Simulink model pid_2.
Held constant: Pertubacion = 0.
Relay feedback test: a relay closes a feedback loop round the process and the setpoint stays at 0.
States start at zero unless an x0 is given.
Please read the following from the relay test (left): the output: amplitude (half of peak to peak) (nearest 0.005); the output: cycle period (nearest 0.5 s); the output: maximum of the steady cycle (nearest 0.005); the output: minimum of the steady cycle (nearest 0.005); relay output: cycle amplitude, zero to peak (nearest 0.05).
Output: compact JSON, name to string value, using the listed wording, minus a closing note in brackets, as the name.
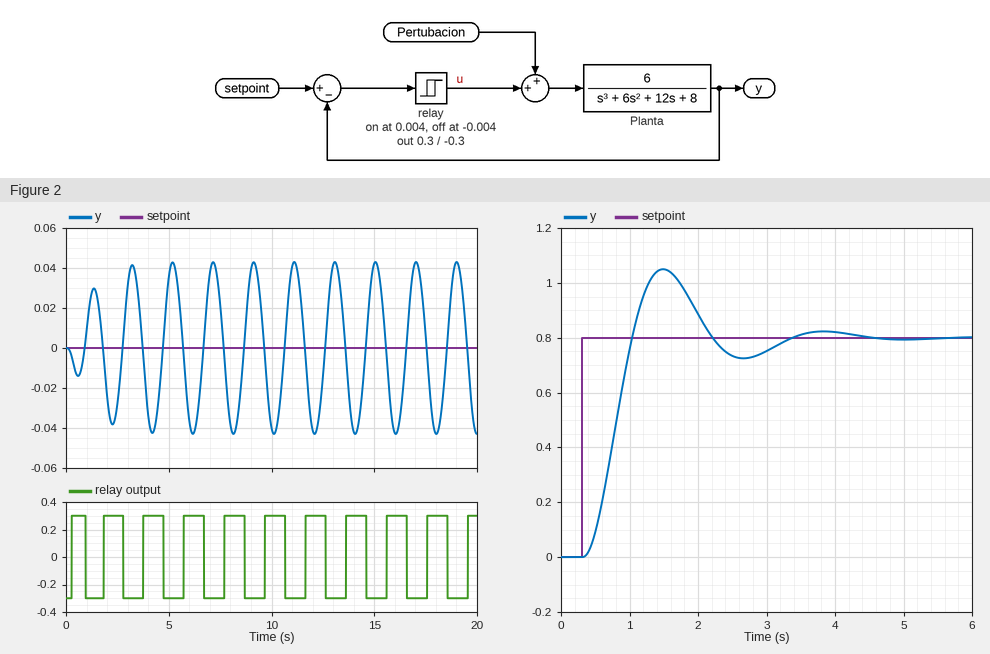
{"the output: amplitude (half of peak to peak)": "0.045", "the output: cycle period": "2.0 s", "the output: maximum of the steady cycle": "0.045", "the output: minimum of the steady cycle": "-0.045", "relay output: cycle amplitude, zero to peak": "0.30"}
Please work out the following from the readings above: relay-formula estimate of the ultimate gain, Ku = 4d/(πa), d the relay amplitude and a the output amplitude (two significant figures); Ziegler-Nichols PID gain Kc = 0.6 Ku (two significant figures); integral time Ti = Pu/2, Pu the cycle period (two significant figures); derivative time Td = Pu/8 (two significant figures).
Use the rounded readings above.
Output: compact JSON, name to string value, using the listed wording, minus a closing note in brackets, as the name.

{"relay-formula estimate of the ultimate gain, Ku = 4d/(πa), d the relay amplitude and a the output amplitude": "8.5", "Ziegler-Nichols PID gain Kc = 0.6 Ku": "5.1", "integral time Ti = Pu/2, Pu the cycle period": "1.0 s", "derivative time Td = Pu/8": "0.25 s"}
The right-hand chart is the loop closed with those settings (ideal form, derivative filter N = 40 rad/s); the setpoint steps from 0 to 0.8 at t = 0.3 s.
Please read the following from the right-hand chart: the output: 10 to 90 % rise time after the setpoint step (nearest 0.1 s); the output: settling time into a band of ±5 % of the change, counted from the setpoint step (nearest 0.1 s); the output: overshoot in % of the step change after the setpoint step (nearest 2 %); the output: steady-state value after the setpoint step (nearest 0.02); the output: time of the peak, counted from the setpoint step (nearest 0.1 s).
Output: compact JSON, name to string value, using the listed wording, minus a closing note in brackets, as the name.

{"the output: 10 to 90 % rise time after the setpoint step": "0.5 s", "the output: settling time into a band of ±5 % of the change, counted from the setpoint step": "2.8 s", "the output: overshoot in % of the step change after the setpoint step": "32 %", "the output: steady-state value after the setpoint step": "0.80", "the output: time of the peak, counted from the setpoint step": "1.2 s"}
